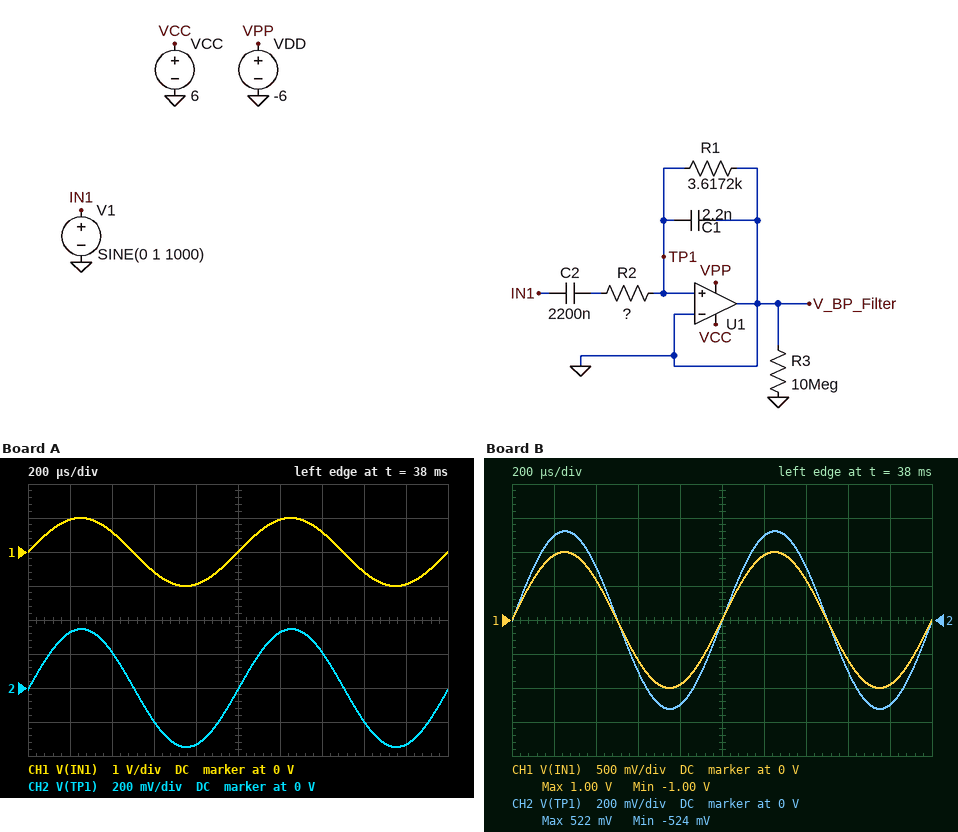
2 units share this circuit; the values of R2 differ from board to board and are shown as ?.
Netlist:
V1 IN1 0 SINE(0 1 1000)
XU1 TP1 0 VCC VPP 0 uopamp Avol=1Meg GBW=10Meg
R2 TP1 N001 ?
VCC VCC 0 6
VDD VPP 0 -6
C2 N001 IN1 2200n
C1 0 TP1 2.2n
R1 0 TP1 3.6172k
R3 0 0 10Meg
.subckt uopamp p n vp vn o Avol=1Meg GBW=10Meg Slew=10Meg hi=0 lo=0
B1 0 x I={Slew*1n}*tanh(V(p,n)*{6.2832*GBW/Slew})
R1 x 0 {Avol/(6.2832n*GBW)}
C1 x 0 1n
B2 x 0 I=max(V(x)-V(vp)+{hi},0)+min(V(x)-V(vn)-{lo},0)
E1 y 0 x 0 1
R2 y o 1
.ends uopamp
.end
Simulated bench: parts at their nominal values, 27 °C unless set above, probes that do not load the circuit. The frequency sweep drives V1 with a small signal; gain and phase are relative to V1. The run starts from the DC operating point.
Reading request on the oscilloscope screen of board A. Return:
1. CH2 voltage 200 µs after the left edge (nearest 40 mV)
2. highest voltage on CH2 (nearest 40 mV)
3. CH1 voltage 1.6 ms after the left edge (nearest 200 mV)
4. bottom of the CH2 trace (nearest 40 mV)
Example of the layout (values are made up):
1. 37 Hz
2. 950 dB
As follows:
1. 320 mV
2. 360 mV
3. -600 mV
4. -360 mV
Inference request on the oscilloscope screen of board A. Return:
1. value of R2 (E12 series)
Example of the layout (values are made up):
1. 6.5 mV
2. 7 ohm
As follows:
1. 6.8 kΩ
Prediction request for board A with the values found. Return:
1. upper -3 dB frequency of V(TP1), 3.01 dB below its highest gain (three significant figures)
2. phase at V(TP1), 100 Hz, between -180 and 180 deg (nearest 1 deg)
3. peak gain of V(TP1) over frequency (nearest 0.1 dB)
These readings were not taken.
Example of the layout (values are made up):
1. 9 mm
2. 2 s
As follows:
1. 30.7 kHz
2. 4 deg
3. -9.2 dB
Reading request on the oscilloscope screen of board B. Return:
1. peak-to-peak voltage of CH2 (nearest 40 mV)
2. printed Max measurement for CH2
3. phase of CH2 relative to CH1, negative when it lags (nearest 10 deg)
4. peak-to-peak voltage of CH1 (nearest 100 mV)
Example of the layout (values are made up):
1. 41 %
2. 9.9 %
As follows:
1. 1.04 V
2. 522 mV
3. 0 deg
4. 2.0 V
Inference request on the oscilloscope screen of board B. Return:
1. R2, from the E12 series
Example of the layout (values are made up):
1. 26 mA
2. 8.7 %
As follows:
1. 3.3 kΩ
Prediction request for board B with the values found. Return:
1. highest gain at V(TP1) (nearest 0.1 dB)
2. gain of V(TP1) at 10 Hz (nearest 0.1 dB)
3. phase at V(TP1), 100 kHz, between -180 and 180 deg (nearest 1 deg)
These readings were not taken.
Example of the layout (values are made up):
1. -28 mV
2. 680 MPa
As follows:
1. -5.6 dB
2. -8.8 dB
3. -67 deg
